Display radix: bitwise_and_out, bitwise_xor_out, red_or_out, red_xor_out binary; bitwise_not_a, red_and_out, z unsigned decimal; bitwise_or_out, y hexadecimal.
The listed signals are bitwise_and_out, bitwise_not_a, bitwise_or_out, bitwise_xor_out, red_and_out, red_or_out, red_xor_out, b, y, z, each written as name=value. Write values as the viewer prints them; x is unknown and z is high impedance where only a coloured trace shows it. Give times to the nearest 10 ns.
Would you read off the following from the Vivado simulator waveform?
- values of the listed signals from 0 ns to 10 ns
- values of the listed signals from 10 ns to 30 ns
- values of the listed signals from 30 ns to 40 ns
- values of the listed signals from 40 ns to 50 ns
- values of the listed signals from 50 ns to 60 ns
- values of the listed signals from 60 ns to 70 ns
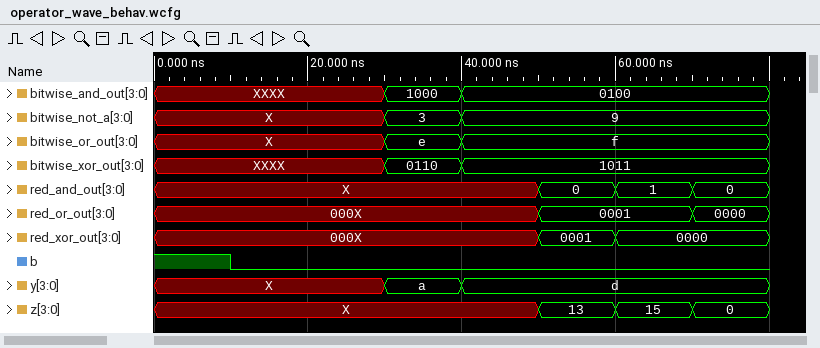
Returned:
bitwise_and_out=XXXX, bitwise_not_a=X, bitwise_or_out=X, bitwise_xor_out=XXXX, red_and_out=X, red_or_out=000X, red_xor_out=000X, b=1, y=X, z=X
bitwise_and_out=XXXX, bitwise_not_a=X, bitwise_or_out=X, bitwise_xor_out=XXXX, red_and_out=X, red_or_out=000X, red_xor_out=000X, b=0, y=X, z=X
bitwise_and_out=1000, bitwise_not_a=3, bitwise_or_out=e, bitwise_xor_out=0110, red_and_out=X, red_or_out=000X, red_xor_out=000X, b=0, y=a, z=X
bitwise_and_out=0100, bitwise_not_a=9, bitwise_or_out=f, bitwise_xor_out=1011, red_and_out=X, red_or_out=000X, red_xor_out=000X, b=0, y=d, z=X
bitwise_and_out=0100, bitwise_not_a=9, bitwise_or_out=f, bitwise_xor_out=1011, red_and_out=0, red_or_out=0001, red_xor_out=0001, b=0, y=d, z=13
bitwise_and_out=0100, bitwise_not_a=9, bitwise_or_out=f, bitwise_xor_out=1011, red_and_out=1, red_or_out=0001, red_xor_out=0000, b=0, y=d, z=15
